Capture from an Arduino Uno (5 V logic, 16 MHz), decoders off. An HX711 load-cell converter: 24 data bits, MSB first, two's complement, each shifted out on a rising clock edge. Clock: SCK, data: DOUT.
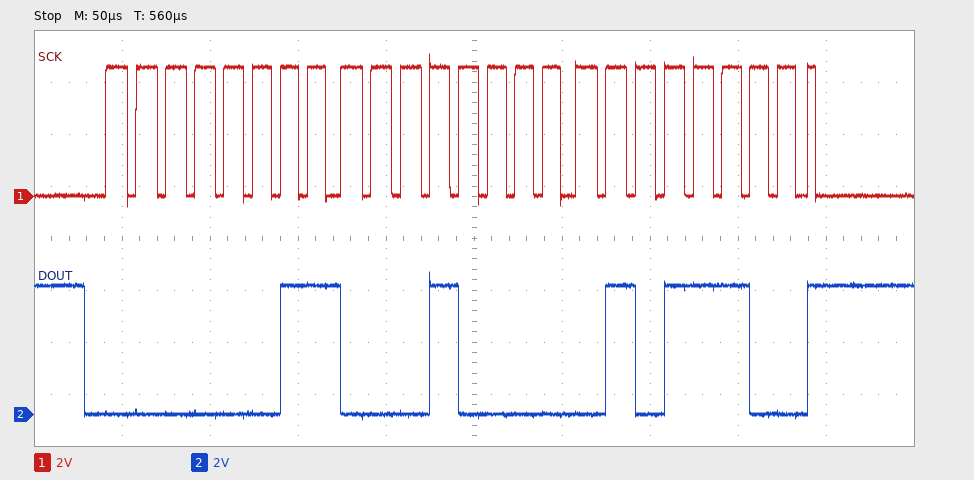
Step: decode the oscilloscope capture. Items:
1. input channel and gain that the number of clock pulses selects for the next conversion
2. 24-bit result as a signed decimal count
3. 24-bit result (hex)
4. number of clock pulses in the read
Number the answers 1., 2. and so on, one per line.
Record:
1. channel A, gain 128
2. 200796
3. 0x03105C
4. 25
